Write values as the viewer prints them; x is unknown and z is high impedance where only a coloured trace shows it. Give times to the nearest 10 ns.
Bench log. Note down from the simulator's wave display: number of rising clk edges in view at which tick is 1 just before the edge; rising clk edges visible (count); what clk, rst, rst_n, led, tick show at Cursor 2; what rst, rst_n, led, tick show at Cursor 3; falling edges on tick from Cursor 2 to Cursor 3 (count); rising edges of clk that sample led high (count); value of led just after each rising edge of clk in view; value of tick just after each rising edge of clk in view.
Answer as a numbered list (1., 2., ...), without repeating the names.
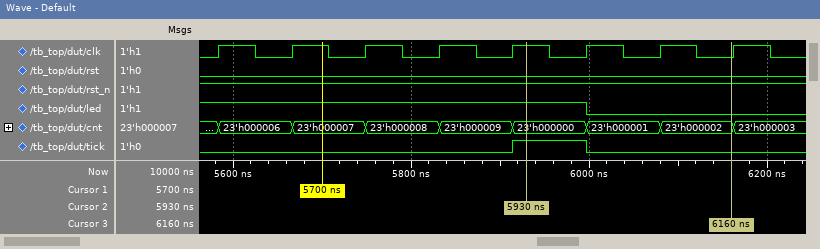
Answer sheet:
1. 1
2. 8
3. clk=1, rst=0, rst_n=1, led=1, tick=1
4. rst=0, rst_n=1, led=0, tick=0
5. 1
6. 6
7. 1 1 1 1 1 0 0 0
8. 0 0 0 0 1 0 0 0
